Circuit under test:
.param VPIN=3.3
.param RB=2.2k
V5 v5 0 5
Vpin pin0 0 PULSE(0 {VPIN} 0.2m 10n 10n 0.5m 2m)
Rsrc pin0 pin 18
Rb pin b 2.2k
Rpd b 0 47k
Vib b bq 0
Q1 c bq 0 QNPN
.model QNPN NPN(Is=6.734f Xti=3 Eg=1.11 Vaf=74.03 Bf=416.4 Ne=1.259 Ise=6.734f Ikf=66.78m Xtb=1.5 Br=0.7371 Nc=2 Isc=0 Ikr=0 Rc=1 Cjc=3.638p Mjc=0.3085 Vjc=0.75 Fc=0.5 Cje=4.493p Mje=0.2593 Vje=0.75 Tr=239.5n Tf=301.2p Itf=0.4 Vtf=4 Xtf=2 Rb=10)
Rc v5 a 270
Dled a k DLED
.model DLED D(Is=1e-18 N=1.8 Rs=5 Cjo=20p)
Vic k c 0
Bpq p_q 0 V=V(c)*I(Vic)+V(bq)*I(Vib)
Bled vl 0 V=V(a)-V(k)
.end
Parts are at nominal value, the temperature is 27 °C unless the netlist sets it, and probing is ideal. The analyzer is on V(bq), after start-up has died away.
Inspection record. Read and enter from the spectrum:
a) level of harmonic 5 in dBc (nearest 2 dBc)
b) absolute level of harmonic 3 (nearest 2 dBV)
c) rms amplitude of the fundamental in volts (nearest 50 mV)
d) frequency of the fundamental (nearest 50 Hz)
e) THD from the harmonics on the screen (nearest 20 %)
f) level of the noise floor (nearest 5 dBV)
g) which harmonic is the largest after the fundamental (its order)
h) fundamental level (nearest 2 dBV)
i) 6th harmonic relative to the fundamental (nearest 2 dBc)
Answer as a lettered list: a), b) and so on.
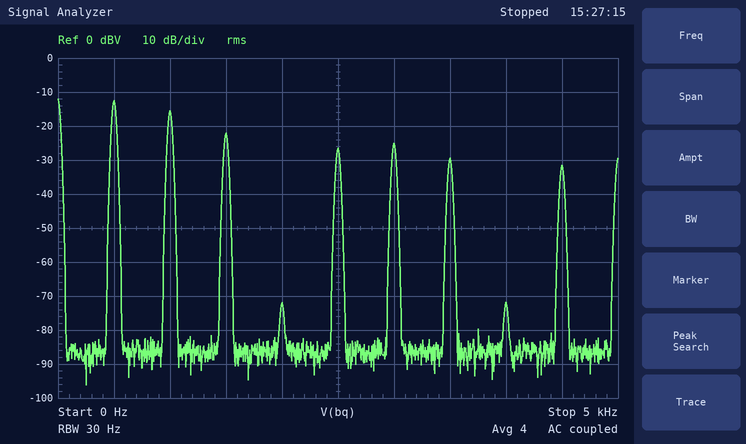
a) -14 dBc
b) -22 dBV
c) 250 mV
d) 500 Hz
e) 80 %
f) -85 dBV
g) 2
h) -12 dBV
i) -12 dBc
